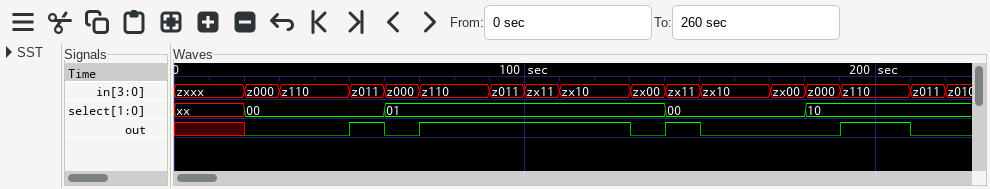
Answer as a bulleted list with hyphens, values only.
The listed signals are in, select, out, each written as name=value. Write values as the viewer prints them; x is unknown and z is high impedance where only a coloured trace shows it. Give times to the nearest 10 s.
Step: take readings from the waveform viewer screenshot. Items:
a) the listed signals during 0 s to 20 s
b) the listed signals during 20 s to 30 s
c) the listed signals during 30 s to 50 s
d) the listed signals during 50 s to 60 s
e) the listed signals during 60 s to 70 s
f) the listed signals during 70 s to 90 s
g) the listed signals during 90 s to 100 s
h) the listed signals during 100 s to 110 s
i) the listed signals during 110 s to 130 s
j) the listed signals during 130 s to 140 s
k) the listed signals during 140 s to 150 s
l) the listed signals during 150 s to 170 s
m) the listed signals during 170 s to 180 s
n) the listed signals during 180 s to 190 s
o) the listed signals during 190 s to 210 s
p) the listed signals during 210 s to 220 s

- in=zxxx, select=xx, out=x
- in=z000, select=00, out=0
- in=z110, select=00, out=0
- in=z011, select=00, out=1
- in=z000, select=01, out=0
- in=z110, select=01, out=1
- in=z011, select=01, out=1
- in=zx11, select=01, out=1
- in=zx10, select=01, out=1
- in=zx00, select=01, out=0
- in=zx11, select=00, out=1
- in=zx10, select=00, out=0
- in=zx00, select=00, out=0
- in=z000, select=10, out=0
- in=z110, select=10, out=1
- in=z011, select=10, out=0
